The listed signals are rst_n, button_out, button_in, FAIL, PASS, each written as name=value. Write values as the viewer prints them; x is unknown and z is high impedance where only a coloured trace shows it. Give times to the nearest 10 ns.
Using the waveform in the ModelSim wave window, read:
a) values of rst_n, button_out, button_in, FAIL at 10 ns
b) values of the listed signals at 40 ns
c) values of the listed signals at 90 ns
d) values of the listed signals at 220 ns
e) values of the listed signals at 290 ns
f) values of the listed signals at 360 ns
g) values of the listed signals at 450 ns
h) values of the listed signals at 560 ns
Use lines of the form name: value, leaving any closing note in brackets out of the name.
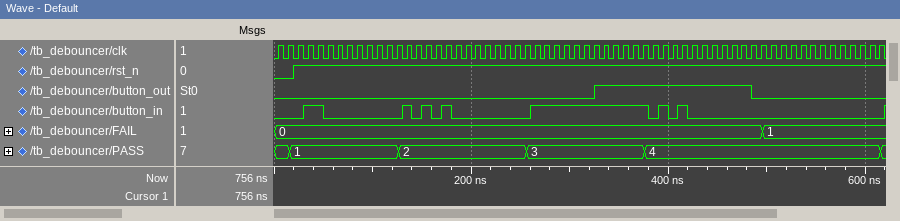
values of rst_n, button_out, button_in, FAIL at 10 ns: rst_n=0, button_out=0, button_in=0, FAIL=0
values of the listed signals at 40 ns: rst_n=1, button_out=0, button_in=1, FAIL=0, PASS=1
values of the listed signals at 90 ns: rst_n=1, button_out=0, button_in=0, FAIL=0, PASS=1
values of the listed signals at 220 ns: rst_n=1, button_out=0, button_in=0, FAIL=0, PASS=2
values of the listed signals at 290 ns: rst_n=1, button_out=0, button_in=1, FAIL=0, PASS=3
values of the listed signals at 360 ns: rst_n=1, button_out=1, button_in=1, FAIL=0, PASS=3
values of the listed signals at 450 ns: rst_n=1, button_out=1, button_in=0, FAIL=0, PASS=4
values of the listed signals at 560 ns: rst_n=1, button_out=0, button_in=0, FAIL=1, PASS=4
